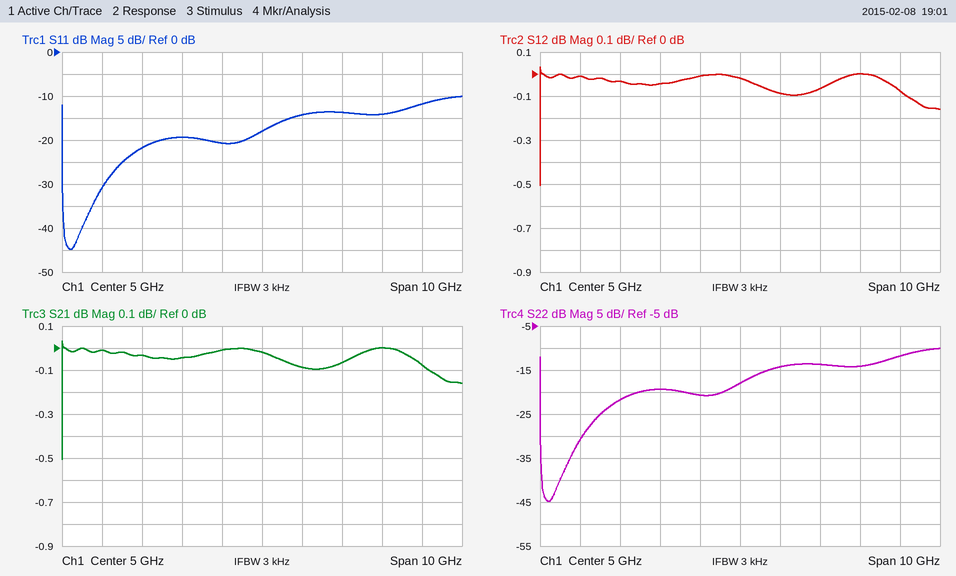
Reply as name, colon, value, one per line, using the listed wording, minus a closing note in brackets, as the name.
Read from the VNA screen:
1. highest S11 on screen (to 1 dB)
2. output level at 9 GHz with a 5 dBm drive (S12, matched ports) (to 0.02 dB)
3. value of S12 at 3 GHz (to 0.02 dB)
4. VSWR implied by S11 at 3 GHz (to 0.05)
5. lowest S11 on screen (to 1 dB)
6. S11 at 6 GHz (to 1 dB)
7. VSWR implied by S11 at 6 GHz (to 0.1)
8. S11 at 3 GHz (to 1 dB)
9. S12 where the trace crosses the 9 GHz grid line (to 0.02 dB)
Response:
highest S11 on screen: -10 dB
output level at 9 GHz with a 5 dBm drive (S12, matched ports): 4.92 dBm
value of S12 at 3 GHz: -0.04 dB
VSWR implied by S11 at 3 GHz: 1.25
lowest S11 on screen: -45 dB
S11 at 6 GHz: -14 dB
VSWR implied by S11 at 6 GHz: 1.5
S11 at 3 GHz: -19 dB
S12 where the trace crosses the 9 GHz grid line: -0.08 dB
